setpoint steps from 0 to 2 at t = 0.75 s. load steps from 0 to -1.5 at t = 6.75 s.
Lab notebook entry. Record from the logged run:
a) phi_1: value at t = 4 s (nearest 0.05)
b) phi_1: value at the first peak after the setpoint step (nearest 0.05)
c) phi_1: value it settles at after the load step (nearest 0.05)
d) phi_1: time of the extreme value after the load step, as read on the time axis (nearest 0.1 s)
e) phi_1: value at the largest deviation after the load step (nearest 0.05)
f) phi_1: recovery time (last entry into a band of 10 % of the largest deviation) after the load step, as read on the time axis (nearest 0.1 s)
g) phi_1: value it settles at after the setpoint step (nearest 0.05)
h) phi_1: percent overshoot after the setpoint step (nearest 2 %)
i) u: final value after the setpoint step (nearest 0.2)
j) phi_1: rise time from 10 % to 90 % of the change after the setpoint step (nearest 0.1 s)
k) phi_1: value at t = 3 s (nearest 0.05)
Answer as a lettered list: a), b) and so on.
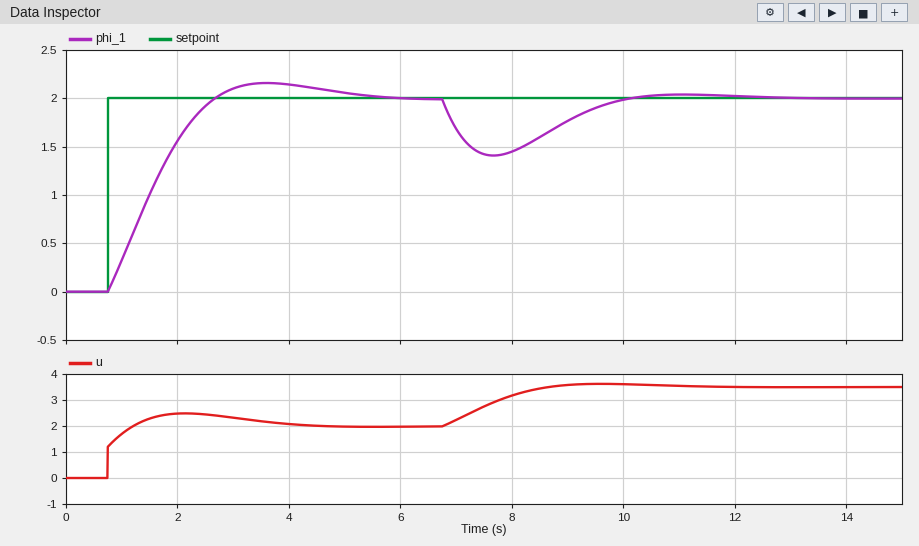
a) 2.15
b) 2.15
c) 2.00
d) 7.7 s
e) 1.40
f) 9.7 s
g) 2.00
h) 8 %
i) 2.0
j) 1.4 s
k) 2.10
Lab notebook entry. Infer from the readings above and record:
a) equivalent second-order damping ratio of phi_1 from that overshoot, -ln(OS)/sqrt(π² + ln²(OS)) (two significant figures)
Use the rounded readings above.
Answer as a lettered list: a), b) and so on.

a) 0.63
